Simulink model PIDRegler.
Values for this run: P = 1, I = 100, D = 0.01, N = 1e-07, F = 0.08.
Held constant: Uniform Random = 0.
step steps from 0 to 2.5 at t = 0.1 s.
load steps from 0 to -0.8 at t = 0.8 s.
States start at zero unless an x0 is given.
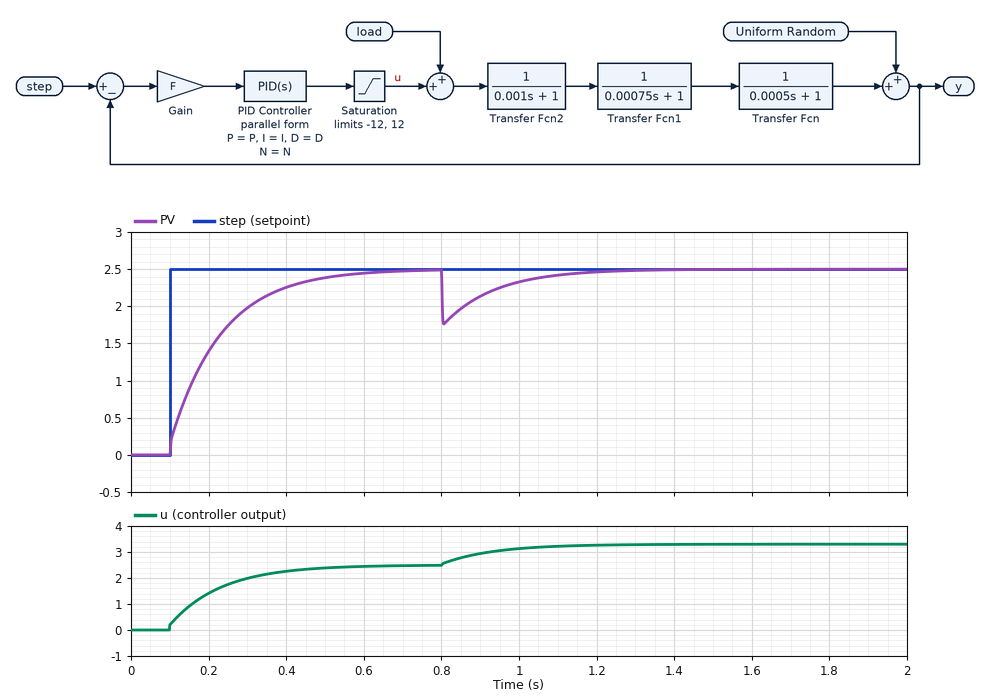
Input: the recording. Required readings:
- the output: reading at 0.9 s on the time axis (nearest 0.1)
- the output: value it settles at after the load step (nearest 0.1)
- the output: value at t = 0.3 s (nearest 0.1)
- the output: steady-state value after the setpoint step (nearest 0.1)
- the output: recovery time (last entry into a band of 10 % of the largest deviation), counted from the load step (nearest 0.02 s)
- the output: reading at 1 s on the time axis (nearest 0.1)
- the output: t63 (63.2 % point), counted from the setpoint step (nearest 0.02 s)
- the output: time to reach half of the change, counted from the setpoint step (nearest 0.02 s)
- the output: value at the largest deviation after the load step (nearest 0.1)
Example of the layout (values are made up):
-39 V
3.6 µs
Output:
2.1
2.5
2.0
2.5
0.32 s
2.3
0.12 s
0.08 s
1.8
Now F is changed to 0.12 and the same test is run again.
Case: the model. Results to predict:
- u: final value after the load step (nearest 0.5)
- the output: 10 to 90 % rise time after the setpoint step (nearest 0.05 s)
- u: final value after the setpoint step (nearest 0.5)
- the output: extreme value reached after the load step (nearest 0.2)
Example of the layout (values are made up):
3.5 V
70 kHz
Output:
3.5
0.20 s
2.5
1.8
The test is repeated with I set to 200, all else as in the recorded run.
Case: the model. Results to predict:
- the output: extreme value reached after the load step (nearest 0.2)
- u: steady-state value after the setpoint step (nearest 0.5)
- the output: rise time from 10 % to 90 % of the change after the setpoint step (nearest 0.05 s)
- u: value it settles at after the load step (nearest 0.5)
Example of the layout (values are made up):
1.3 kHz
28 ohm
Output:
1.8
2.5
0.15 s
3.5
